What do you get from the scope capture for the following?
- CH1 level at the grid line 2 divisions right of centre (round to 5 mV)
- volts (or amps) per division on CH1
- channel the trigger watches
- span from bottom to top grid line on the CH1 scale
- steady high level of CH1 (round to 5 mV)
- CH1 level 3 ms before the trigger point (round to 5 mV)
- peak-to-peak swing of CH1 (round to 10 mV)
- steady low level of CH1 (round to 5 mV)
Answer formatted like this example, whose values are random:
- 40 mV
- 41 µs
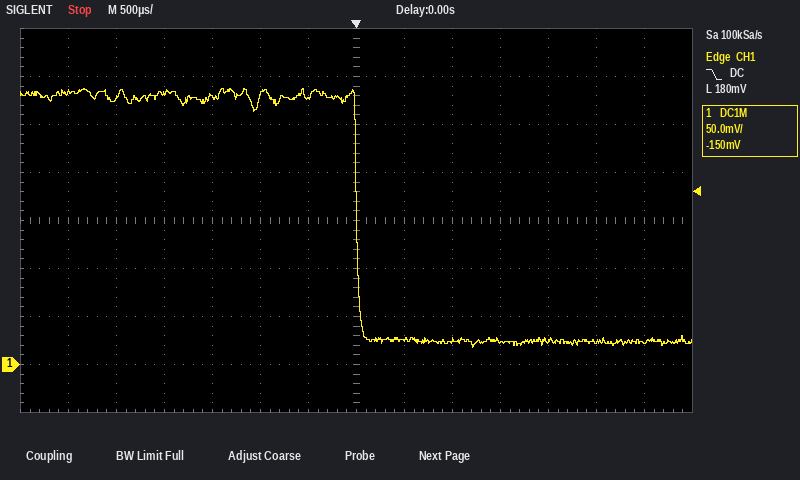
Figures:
- 25 mV
- 50 mV
- CH1
- 400 mV
- 280 mV
- 285 mV
- 270 mV
- 25 mV
